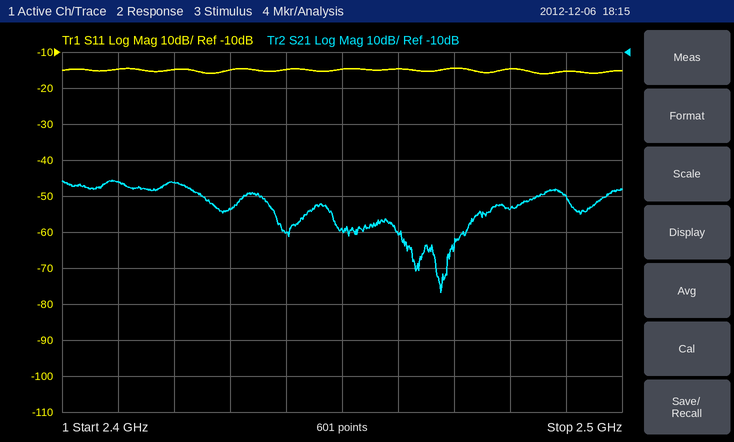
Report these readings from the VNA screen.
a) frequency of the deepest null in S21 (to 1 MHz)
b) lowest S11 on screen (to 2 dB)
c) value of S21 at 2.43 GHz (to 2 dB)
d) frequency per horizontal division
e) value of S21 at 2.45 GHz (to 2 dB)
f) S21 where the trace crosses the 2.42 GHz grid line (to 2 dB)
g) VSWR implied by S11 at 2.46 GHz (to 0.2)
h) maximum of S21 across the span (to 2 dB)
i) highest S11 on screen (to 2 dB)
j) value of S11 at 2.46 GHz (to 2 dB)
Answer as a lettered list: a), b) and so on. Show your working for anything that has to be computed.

a) 2.468 GHz
b) -16 dB
c) -54 dB
d) 10 MHz
e) -60 dB
f) -46 dB
g) |Γ| = 10^(-14/20) = 0.1995; VSWR = (1 + 0.1995)/(1 − 0.1995) ≈ 1.50, so 1.4 to the nearest 0.2
h) -46 dB
i) -14 dB
j) -14 dB
